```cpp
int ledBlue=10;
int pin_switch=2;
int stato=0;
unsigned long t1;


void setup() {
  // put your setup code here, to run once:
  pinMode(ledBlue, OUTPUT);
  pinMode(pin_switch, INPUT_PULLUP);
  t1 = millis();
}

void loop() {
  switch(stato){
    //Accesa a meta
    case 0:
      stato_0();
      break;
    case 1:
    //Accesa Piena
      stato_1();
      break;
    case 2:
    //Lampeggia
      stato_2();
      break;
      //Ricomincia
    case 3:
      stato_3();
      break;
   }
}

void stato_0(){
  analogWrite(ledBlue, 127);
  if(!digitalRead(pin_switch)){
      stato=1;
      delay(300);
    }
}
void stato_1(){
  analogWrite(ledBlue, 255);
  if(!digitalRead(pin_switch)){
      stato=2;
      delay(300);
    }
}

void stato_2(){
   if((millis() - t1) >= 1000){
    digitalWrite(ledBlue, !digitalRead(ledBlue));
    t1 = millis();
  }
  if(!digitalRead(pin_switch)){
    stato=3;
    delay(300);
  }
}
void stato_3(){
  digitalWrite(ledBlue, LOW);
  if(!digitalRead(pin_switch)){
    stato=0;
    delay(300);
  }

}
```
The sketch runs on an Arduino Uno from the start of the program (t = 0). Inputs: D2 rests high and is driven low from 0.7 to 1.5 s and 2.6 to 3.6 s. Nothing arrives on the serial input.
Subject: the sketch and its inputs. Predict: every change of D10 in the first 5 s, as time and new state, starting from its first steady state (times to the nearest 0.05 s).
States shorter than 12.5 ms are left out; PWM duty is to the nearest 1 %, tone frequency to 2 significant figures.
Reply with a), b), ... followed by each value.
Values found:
a) 0 s PWM 50 %; 1 s high; 1.3 s low; 2.9 s PWM 50 %; 3.2 s high; 3.5 s low
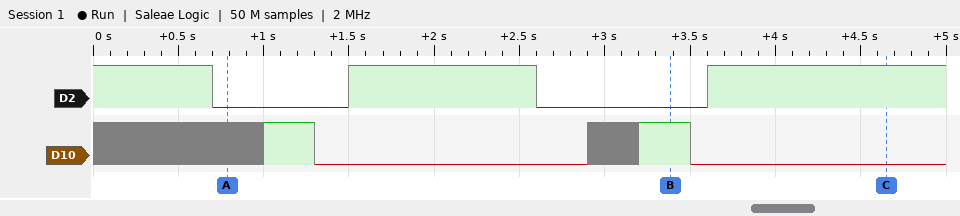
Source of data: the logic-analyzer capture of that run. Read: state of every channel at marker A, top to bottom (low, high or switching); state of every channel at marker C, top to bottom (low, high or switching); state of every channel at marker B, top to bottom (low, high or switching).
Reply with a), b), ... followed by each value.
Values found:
a) D2 low, D10 switching
b) D2 high, D10 low
c) D2 low, D10 high
